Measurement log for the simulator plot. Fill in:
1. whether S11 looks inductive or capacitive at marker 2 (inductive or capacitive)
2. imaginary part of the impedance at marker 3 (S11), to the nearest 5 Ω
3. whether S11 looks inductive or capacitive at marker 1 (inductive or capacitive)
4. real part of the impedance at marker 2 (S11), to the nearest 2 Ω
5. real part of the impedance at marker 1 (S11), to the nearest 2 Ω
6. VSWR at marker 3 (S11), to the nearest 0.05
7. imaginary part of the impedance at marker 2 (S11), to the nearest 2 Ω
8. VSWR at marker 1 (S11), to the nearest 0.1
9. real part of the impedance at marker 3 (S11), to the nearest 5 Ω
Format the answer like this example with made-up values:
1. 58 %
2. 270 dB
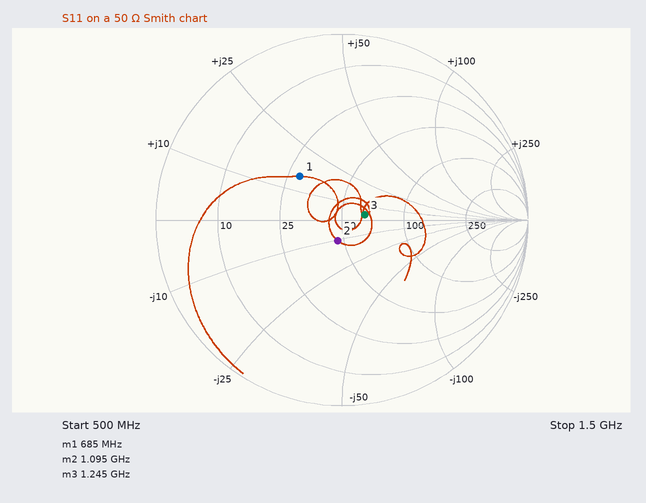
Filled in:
1. capacitive
2. +5 Ω
3. inductive
4. 46 Ω
5. 28 Ω
6. 1.30
7. -10 Ω
8. 2.0
9. 65 Ω
